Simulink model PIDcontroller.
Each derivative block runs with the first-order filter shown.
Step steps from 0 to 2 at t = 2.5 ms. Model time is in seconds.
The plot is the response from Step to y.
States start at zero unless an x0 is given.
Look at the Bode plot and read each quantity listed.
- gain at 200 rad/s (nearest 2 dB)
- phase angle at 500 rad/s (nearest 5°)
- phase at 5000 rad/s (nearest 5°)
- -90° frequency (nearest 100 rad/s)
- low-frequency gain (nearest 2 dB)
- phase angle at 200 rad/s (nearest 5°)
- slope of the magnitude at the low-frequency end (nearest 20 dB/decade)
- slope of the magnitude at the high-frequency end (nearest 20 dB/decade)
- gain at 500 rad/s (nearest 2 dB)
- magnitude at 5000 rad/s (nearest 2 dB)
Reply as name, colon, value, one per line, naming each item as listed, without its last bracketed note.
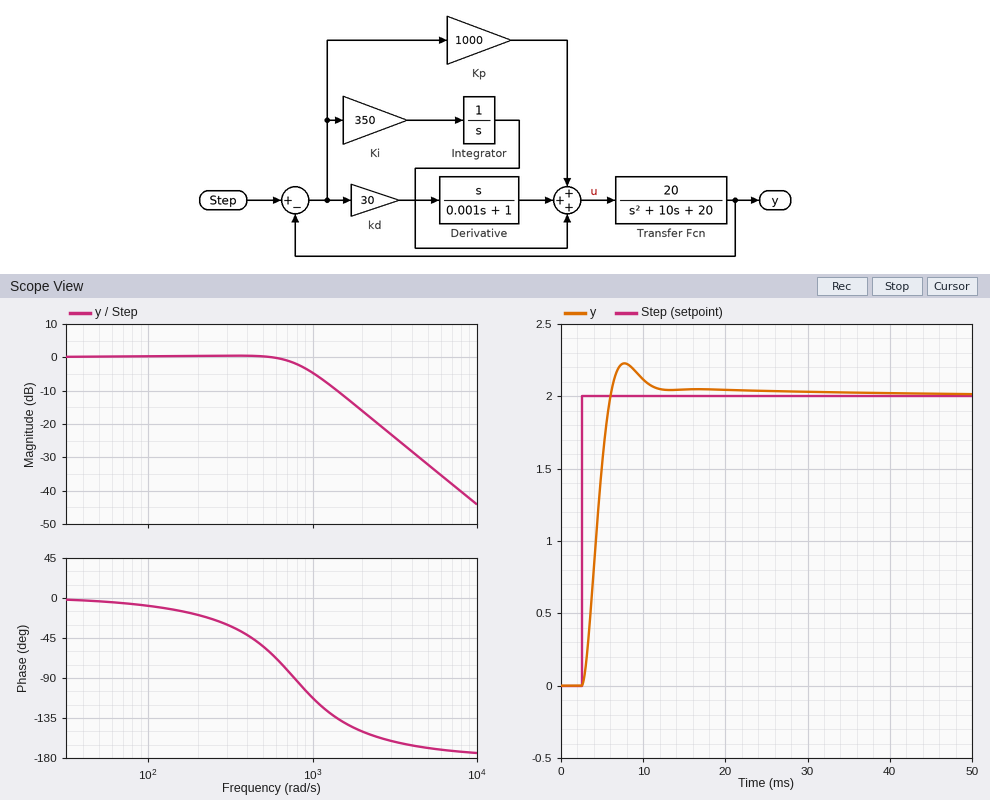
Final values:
gain at 200 rad/s: 0 dB
phase angle at 500 rad/s: -55°
phase at 5000 rad/s: -170°
-90° frequency: 800 rad/s
low-frequency gain: 0 dB
phase angle at 200 rad/s: -20°
slope of the magnitude at the low-frequency end: 0 dB/decade
slope of the magnitude at the high-frequency end: -40 dB/decade
gain at 500 rad/s: 0 dB
magnitude at 5000 rad/s: -32 dB
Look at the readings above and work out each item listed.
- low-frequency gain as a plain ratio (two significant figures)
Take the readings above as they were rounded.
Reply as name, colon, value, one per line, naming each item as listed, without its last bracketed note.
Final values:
low-frequency gain as a plain ratio: 1.0
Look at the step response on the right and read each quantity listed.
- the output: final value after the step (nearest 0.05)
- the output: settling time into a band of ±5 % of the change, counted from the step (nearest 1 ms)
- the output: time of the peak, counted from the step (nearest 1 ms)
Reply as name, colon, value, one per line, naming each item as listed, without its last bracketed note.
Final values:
the output: final value after the step: 2.00
the output: settling time into a band of ±5 % of the change, counted from the step: 8 ms
the output: time of the peak, counted from the step: 5 ms
